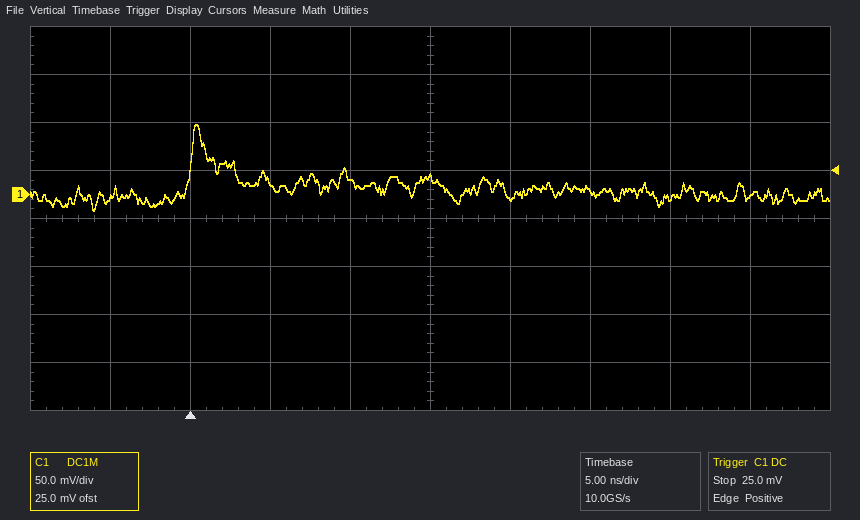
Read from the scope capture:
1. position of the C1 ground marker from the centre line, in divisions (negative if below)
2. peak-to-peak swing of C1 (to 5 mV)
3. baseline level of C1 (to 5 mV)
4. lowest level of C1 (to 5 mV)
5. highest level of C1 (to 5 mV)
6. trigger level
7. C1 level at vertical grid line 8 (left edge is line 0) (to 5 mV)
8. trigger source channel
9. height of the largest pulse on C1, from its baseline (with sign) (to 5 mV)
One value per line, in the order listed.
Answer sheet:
+0.5 div
90 mV
5 mV
-15 mV
75 mV
25.0 mV
-5 mV
C1
+70 mV
